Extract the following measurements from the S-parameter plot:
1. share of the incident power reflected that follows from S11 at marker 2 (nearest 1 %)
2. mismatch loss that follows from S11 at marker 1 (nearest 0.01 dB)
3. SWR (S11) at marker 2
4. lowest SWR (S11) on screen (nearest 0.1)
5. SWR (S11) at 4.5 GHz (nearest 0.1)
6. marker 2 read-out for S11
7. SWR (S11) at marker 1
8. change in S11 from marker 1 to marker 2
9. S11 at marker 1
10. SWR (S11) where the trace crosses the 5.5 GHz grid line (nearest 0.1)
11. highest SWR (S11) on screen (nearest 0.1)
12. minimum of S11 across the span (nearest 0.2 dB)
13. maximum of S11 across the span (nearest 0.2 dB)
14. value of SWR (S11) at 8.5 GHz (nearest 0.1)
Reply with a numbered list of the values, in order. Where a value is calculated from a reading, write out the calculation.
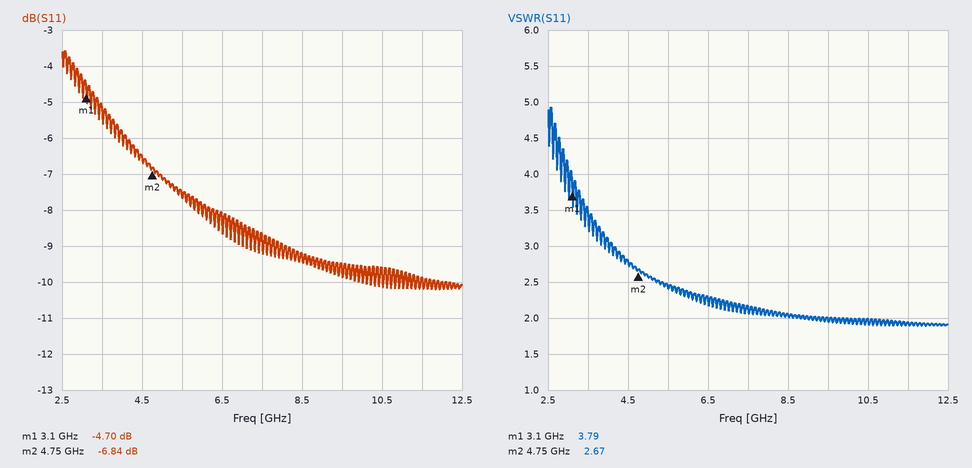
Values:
1. 10^(-6.84/10) ≈ 21 %
2. −10 log10(1 − 10^(-4.7/10)) ≈ 1.80 dB
3. 2.67
4. 1.9
5. 2.8
6. -6.84 dB
7. 3.79
8. -6.84 − (-4.7) = -2.14 dB
9. -4.70 dB
10. 2.4
11. 4.9
12. -10.2 dB
13. -3.6 dB
14. 2.0
